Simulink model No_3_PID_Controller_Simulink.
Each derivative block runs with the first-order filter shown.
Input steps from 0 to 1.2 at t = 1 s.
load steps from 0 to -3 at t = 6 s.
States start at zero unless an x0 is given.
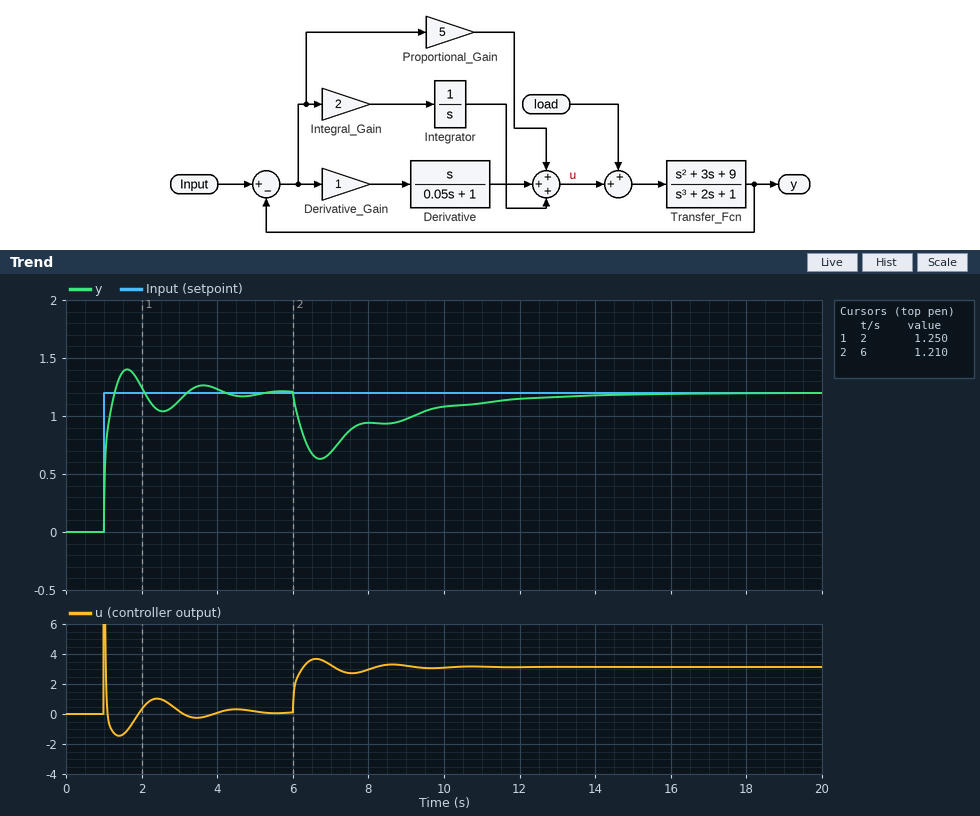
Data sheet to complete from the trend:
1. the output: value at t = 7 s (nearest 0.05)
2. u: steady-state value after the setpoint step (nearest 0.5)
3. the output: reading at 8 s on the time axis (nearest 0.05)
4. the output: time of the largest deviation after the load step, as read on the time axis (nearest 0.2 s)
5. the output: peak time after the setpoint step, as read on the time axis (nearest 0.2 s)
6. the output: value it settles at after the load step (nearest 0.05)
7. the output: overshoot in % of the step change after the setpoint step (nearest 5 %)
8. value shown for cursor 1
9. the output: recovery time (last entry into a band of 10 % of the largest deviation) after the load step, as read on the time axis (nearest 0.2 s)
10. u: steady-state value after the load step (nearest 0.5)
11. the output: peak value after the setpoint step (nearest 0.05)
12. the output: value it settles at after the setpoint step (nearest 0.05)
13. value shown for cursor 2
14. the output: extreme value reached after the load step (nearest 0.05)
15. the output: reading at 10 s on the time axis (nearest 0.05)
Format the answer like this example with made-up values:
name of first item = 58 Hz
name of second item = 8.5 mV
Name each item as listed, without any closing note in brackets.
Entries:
the output: value at t = 7 s = 0.70
u: steady-state value after the setpoint step = 0.0
the output: reading at 8 s on the time axis = 0.95
the output: time of the largest deviation after the load step, as read on the time axis = 6.8 s
the output: peak time after the setpoint step, as read on the time axis = 1.6 s
the output: value it settles at after the load step = 1.20
the output: overshoot in % of the step change after the setpoint step = 15 %
value shown for cursor 1 = 1.250
the output: recovery time (last entry into a band of 10 % of the largest deviation) after the load step, as read on the time axis = 11.8 s
u: steady-state value after the load step = 3.0
the output: peak value after the setpoint step = 1.40
the output: value it settles at after the setpoint step = 1.20
value shown for cursor 2 = 1.210
the output: extreme value reached after the load step = 0.65
the output: reading at 10 s on the time axis = 1.10
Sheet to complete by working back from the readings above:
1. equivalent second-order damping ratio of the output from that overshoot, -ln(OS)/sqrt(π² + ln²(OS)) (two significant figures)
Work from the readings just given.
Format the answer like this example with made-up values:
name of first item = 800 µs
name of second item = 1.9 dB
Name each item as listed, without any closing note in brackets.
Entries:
equivalent second-order damping ratio of the output from that overshoot, -ln(OS)/sqrt(π² + ln²(OS)) = 0.52
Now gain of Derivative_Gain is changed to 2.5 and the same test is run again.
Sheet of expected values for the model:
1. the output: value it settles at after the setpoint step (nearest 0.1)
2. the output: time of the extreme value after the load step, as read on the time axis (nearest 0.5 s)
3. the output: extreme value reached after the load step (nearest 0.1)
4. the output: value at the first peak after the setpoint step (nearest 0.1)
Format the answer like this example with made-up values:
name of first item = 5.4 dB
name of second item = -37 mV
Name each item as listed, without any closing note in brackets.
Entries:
the output: value it settles at after the setpoint step = 1.2
the output: time of the extreme value after the load step, as read on the time axis = 7.0 s
the output: extreme value reached after the load step = 0.7
the output: value at the first peak after the setpoint step = 1.3
